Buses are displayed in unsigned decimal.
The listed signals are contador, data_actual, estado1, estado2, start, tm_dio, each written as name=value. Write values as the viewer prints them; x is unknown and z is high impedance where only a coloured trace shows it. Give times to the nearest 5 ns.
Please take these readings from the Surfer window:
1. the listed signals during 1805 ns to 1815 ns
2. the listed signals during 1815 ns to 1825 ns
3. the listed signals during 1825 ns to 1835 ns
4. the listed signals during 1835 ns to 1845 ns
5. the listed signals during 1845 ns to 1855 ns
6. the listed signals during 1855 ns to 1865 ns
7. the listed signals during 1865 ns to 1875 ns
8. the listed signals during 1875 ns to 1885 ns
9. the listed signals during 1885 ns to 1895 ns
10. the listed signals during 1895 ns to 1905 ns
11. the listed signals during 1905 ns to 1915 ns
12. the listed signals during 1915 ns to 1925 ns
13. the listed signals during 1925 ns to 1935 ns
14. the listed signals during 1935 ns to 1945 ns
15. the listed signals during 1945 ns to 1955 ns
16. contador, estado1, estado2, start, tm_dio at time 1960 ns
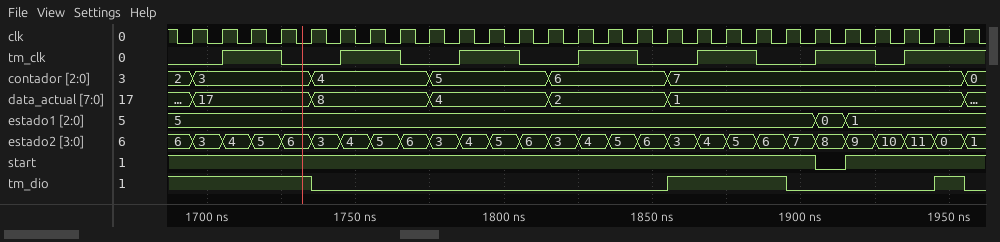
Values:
contador=5, data_actual=4, estado1=5, estado2=6, start=1, tm_dio=0
contador=6, data_actual=2, estado1=5, estado2=3, start=1, tm_dio=0
contador=6, data_actual=2, estado1=5, estado2=4, start=1, tm_dio=0
contador=6, data_actual=2, estado1=5, estado2=5, start=1, tm_dio=0
contador=6, data_actual=2, estado1=5, estado2=6, start=1, tm_dio=0
contador=7, data_actual=1, estado1=5, estado2=3, start=1, tm_dio=1
contador=7, data_actual=1, estado1=5, estado2=4, start=1, tm_dio=1
contador=7, data_actual=1, estado1=5, estado2=5, start=1, tm_dio=1
contador=7, data_actual=1, estado1=5, estado2=6, start=1, tm_dio=1
contador=7, data_actual=1, estado1=5, estado2=7, start=1, tm_dio=0
contador=7, data_actual=1, estado1=0, estado2=8, start=0, tm_dio=0
contador=7, data_actual=1, estado1=1, estado2=9, start=1, tm_dio=0
contador=7, data_actual=1, estado1=1, estado2=10, start=1, tm_dio=0
contador=7, data_actual=1, estado1=1, estado2=11, start=1, tm_dio=0
contador=7, data_actual=1, estado1=1, estado2=0, start=1, tm_dio=1
contador=0, estado1=1, estado2=1, start=1, tm_dio=0
